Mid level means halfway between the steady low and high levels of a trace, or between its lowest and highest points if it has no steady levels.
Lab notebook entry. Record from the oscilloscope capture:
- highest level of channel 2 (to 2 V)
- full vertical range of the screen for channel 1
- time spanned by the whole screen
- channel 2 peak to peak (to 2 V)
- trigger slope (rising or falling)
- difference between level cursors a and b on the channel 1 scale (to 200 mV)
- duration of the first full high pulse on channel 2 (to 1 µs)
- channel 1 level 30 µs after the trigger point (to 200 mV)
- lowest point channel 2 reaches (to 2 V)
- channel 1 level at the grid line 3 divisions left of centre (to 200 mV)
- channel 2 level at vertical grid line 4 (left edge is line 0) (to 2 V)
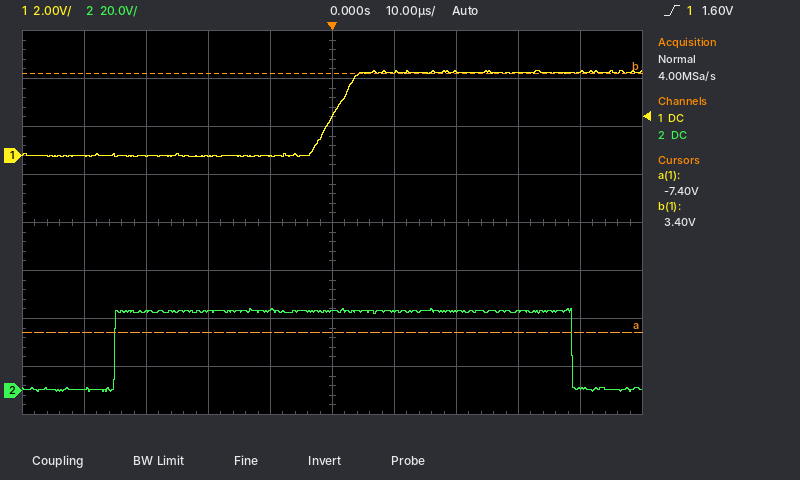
34 V
16 V
100 µs
34 V
rising
10.8 V
74 µs
3.4 V
0 V
0.0 V
34 V
